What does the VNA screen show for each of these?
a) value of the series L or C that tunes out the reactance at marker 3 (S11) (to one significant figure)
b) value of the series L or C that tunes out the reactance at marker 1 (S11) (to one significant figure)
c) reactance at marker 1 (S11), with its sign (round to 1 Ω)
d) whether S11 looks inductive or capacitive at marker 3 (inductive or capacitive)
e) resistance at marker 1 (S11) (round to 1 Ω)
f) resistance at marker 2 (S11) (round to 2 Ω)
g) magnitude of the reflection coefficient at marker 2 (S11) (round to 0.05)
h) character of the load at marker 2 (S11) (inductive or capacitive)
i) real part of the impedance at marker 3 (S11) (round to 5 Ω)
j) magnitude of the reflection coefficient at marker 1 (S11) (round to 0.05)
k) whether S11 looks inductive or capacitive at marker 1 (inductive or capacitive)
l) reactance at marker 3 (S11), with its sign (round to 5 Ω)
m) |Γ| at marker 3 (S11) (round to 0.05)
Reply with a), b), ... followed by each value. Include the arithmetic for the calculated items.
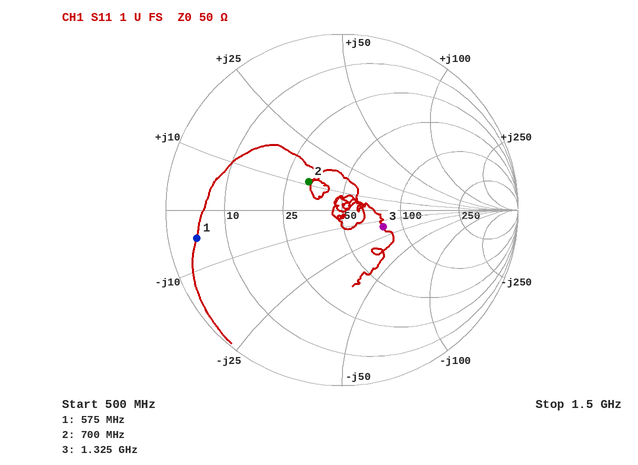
a) L = 15 Ω/(2π × 1.325 GHz) ≈ 2 nH
b) L = 5 Ω/(2π × 575 MHz) ≈ 1 nH
c) -5 Ω
d) capacitive
e) 4 Ω
f) 32 Ω
g) 0.25
h) inductive
i) 80 Ω
j) 0.85
k) capacitive
l) -15 Ω
m) 0.25
